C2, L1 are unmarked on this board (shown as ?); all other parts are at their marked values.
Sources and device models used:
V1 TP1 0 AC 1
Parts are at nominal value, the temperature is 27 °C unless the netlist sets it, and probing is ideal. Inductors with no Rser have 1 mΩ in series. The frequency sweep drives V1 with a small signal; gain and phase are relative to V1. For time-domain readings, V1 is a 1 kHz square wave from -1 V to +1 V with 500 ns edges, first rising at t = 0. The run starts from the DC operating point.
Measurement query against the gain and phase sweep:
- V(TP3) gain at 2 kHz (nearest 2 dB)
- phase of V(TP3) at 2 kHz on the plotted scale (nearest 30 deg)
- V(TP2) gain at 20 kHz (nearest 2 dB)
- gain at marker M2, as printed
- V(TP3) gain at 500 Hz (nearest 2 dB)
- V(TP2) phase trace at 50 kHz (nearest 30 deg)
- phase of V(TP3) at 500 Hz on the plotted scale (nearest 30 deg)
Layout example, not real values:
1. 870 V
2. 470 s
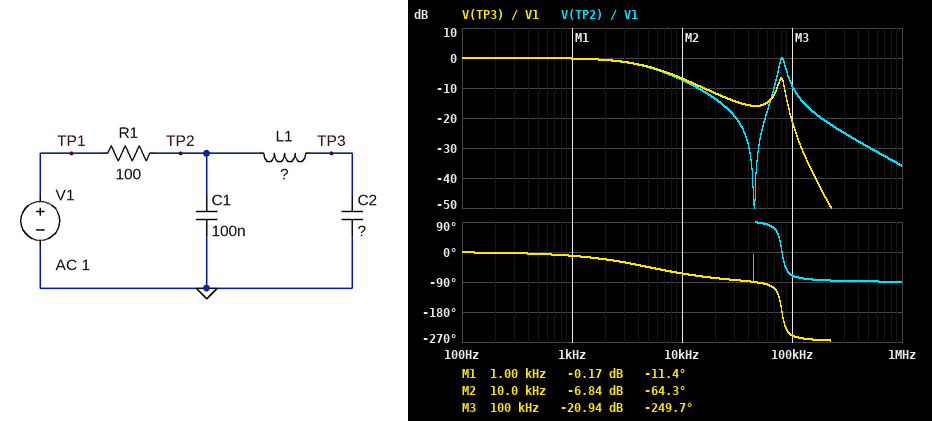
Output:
1. 0 dB
2. -30 deg
3. -14 dB
4. -6.84 dB
5. 0 dB
6. 90 deg
7. 0 deg
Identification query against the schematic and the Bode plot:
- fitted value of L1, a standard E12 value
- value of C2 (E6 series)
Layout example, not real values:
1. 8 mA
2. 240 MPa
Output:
1. 56 µH
2. 220 nF
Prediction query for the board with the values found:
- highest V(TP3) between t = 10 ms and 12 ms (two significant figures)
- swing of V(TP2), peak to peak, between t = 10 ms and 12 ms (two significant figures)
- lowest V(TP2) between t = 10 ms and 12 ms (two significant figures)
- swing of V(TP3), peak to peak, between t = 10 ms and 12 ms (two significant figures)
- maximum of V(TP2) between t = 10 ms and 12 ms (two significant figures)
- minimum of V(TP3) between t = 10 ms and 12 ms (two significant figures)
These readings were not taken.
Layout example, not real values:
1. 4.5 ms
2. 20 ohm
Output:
1. 1.0 V
2. 2.0 V
3. -1.0 V
4. 2.0 V
5. 1.0 V
6. -1.0 V
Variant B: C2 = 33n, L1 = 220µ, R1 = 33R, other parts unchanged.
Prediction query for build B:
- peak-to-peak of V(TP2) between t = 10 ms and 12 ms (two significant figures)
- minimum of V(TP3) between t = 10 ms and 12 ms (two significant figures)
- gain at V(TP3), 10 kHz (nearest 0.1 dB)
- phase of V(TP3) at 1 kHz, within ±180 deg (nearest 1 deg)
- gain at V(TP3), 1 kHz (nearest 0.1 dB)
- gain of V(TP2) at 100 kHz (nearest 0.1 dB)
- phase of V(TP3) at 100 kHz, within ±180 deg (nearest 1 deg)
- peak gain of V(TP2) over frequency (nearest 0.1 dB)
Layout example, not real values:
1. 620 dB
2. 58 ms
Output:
1. 2.3 V
2. -1.7 V
3. -0.1 dB
4. -2 deg
5. 0 dB
6. -5.9 dB
7. 120 deg
8. 0 dB
